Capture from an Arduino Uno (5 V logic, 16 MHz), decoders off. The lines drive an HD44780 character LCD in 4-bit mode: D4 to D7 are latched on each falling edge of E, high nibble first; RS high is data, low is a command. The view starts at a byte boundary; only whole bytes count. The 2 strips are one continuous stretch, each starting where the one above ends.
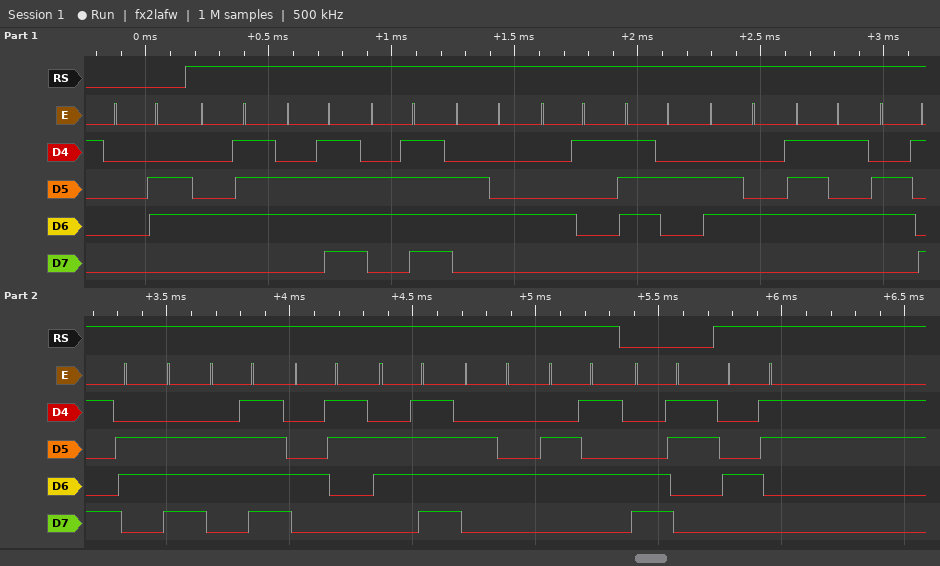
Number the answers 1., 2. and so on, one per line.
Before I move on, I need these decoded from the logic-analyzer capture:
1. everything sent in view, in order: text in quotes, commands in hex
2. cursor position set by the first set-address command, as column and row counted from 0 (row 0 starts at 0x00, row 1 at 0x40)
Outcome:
1. 0x06 "GoodArduinoCode" 0xC3 "C"
2. column 3, row 1
